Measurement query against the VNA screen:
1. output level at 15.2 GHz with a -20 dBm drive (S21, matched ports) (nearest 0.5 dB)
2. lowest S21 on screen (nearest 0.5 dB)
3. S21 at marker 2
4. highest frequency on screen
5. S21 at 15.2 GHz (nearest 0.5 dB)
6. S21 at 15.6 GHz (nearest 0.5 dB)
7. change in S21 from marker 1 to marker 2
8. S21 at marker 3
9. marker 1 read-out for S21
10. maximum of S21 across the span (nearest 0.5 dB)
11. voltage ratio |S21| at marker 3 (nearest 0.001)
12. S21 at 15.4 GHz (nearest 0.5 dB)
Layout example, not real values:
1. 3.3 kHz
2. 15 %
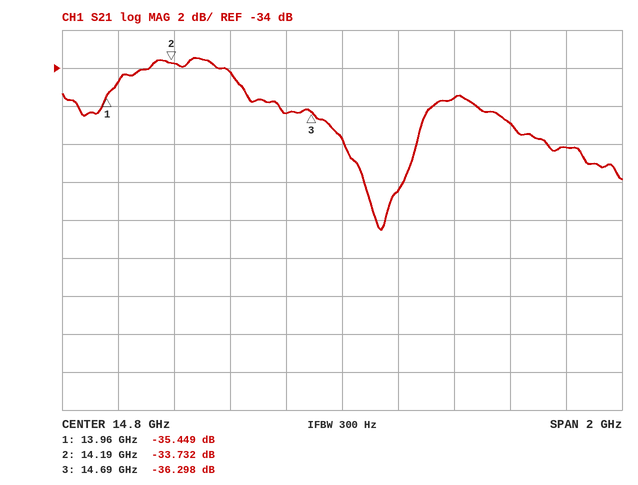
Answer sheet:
1. -55.5 dBm
2. -42.5 dB
3. -33.732 dB
4. 15.8 GHz
5. -35.5 dB
6. -38.0 dB
7. 1.717 dB
8. -36.298 dB
9. -35.449 dB
10. -33.5 dB
11. 0.015
12. -37.0 dB
